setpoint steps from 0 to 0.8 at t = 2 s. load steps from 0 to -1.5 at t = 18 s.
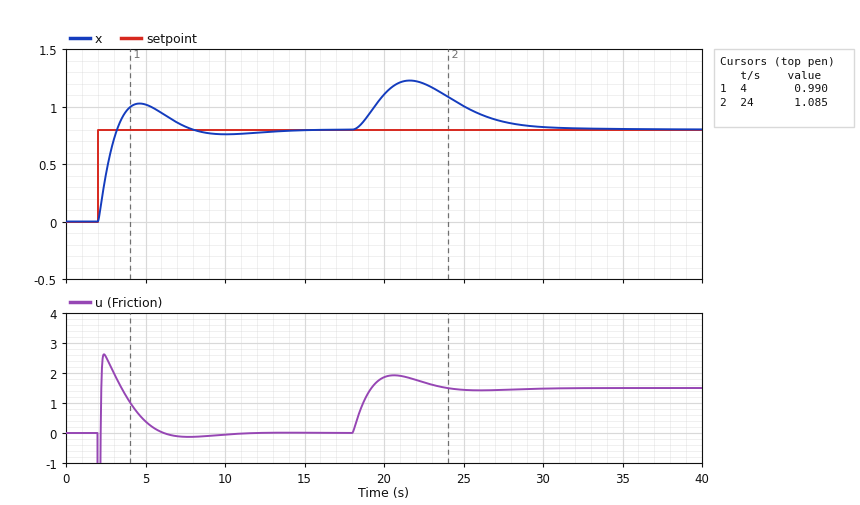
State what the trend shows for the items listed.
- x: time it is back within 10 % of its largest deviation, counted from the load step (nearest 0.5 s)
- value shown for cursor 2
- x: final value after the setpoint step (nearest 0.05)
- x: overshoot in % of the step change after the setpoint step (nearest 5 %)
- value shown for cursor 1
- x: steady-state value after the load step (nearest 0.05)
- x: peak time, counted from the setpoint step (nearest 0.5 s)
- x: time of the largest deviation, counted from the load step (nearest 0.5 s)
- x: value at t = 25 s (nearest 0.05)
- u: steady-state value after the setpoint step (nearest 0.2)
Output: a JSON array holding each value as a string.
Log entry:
["10.5 s", "1.085", "0.80", "30 %", "0.990", "0.80", "2.5 s", "3.5 s", "1.00", "0.0"]
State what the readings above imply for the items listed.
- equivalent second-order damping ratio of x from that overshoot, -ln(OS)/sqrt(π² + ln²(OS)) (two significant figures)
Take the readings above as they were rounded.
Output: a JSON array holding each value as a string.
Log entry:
["0.36"]
